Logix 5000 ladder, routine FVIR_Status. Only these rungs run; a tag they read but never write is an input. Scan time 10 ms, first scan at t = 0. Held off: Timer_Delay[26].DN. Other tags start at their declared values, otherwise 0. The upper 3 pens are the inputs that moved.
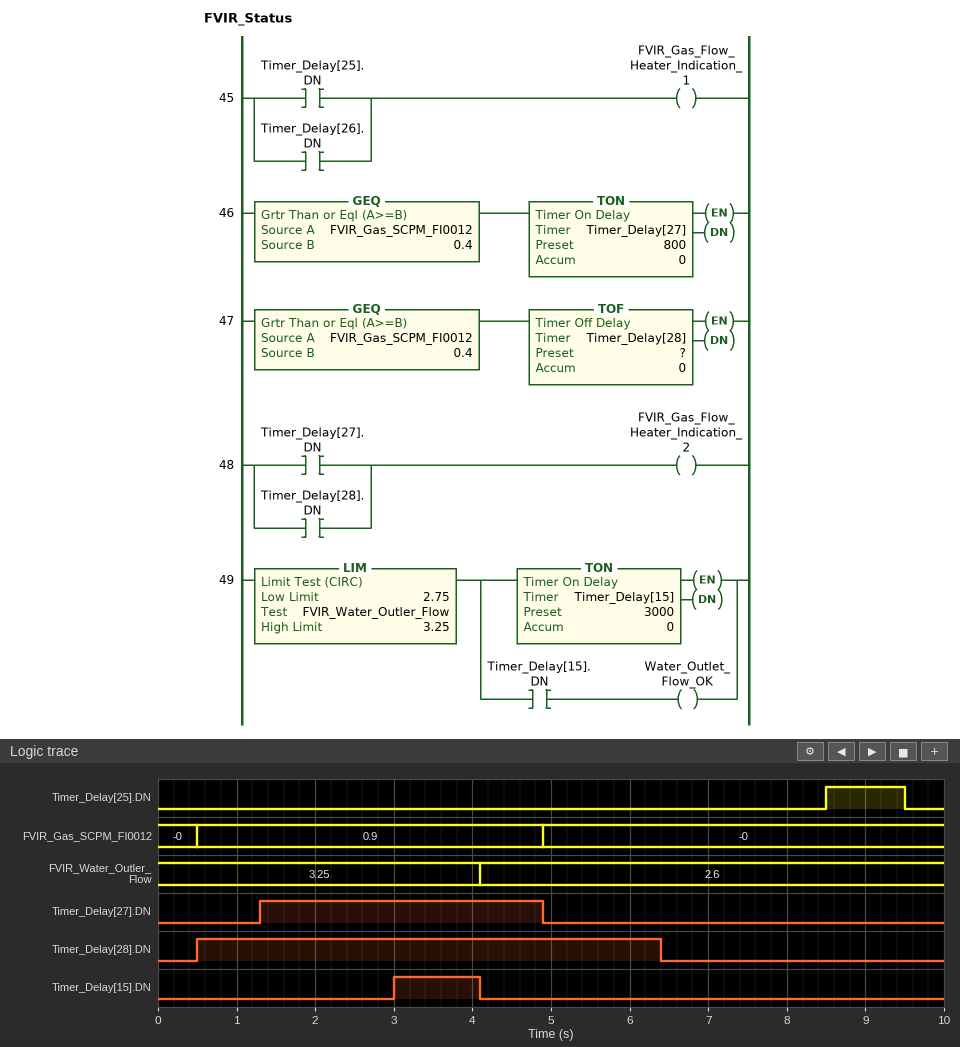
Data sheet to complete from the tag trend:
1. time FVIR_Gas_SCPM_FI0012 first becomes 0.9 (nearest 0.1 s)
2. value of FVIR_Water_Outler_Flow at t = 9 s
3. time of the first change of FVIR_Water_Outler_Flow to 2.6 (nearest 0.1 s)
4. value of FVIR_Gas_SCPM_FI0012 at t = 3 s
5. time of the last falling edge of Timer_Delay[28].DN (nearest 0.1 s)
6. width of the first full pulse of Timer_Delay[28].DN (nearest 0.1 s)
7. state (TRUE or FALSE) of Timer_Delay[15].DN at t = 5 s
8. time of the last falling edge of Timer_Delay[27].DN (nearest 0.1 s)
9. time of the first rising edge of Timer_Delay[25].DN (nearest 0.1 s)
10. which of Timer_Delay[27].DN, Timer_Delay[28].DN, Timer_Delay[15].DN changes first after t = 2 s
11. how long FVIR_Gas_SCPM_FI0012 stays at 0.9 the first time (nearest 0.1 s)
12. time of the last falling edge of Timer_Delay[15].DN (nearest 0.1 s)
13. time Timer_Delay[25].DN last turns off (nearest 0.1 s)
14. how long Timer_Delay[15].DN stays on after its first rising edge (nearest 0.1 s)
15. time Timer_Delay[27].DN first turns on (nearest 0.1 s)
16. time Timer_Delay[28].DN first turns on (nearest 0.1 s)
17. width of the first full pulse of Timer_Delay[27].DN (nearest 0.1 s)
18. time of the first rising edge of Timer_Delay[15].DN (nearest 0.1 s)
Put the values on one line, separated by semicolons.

0.5 s; 2.6; 4.1 s; 0.9; 6.4 s; 5.9 s; FALSE; 4.9 s; 8.5 s; Timer_Delay[15].DN; 4.4 s; 4.1 s; 9.5 s; 1.1 s; 1.3 s; 0.5 s; 3.6 s; 3.0 s
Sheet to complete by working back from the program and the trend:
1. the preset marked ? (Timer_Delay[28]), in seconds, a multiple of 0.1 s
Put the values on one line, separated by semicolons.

1.5 s
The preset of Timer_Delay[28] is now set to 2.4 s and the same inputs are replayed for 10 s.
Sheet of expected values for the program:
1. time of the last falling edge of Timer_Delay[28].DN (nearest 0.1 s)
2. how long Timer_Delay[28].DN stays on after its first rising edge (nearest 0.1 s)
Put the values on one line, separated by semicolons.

7.3 s; 6.8 s
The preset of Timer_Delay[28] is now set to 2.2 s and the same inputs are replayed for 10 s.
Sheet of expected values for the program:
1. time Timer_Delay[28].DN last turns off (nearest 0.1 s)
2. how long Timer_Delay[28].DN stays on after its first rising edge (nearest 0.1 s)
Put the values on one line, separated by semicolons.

7.1 s; 6.6 s
